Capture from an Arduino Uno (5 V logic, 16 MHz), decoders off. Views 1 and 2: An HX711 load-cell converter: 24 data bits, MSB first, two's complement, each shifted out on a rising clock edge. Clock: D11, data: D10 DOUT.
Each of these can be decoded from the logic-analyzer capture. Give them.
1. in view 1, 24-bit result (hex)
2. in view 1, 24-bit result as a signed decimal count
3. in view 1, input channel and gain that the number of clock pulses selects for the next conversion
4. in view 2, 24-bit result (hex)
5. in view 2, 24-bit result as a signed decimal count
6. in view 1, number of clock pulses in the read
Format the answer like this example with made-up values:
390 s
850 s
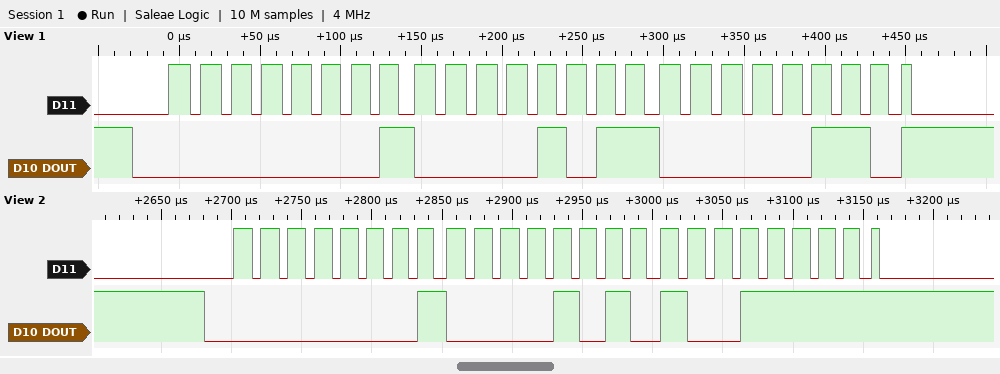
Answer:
0x010B06
68358
channel A, gain 128
0x010A9F
68255
25
